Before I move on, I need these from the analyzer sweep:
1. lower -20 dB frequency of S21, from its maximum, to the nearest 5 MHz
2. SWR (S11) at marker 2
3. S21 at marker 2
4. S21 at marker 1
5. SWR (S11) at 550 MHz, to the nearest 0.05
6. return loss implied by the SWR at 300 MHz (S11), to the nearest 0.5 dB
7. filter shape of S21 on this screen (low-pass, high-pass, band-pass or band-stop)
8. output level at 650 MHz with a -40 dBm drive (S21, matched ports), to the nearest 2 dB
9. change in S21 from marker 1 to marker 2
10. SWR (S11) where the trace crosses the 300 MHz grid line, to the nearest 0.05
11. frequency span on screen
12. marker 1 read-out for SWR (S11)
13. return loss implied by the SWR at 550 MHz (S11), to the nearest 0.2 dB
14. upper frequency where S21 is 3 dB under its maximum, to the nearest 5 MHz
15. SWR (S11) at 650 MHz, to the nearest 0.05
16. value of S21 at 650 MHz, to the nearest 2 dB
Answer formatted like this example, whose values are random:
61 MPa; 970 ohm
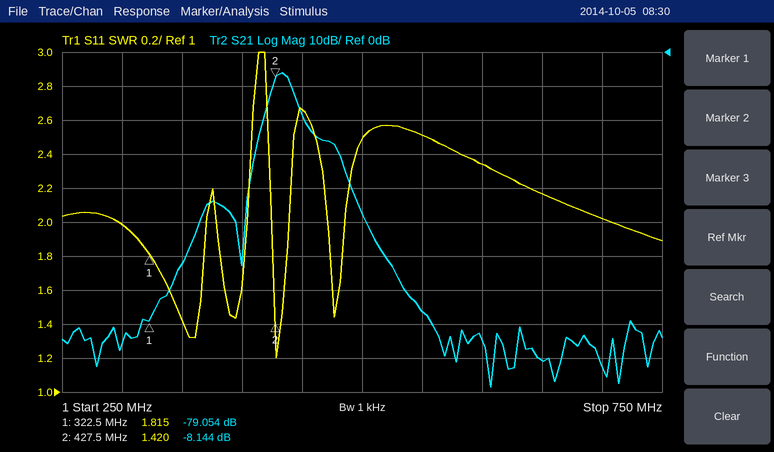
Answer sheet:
415 MHz; 1.420; -8.144 dB; -79.054 dB; 2.50; 9.5 dB; band-pass; -130 dBm; 70.910 dB; 2.00; 500 MHz; 1.815; 7.4 dB; 440 MHz; 2.15; -90 dB
